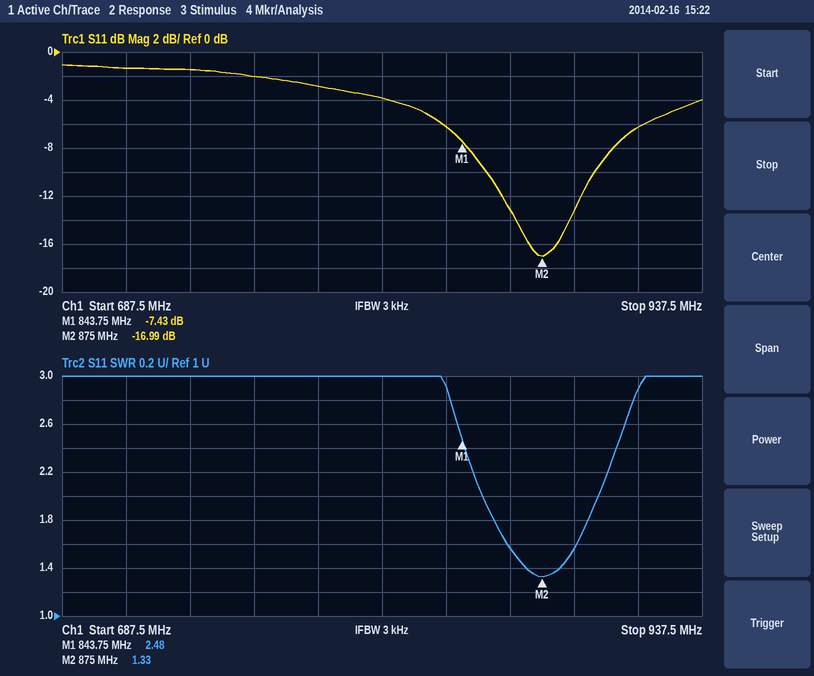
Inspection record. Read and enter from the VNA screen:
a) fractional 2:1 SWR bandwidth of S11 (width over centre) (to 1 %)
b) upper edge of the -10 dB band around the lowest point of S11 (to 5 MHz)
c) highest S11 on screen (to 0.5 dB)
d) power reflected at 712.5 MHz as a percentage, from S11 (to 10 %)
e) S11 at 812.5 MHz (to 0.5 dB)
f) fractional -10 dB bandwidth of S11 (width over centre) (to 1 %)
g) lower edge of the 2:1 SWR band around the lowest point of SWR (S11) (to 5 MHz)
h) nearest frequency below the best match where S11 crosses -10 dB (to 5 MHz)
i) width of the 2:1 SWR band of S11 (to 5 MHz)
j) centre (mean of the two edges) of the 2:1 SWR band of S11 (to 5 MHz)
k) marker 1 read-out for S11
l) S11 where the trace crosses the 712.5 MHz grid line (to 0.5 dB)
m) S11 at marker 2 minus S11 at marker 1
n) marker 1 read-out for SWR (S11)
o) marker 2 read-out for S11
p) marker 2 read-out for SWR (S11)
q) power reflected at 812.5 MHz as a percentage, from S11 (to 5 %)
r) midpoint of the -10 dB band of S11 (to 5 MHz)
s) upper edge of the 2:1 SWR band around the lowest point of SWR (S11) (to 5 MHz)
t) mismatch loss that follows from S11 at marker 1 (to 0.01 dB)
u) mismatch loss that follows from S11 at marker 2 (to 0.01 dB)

5 %
895 MHz
-1.0 dB
70 %
-4.0 dB
5 %
850 MHz
855 MHz
45 MHz
875 MHz
-7.43 dB
-1.5 dB
-9.56 dB
2.48
-16.99 dB
1.33
40 %
875 MHz
895 MHz
0.87 dB
0.09 dB
